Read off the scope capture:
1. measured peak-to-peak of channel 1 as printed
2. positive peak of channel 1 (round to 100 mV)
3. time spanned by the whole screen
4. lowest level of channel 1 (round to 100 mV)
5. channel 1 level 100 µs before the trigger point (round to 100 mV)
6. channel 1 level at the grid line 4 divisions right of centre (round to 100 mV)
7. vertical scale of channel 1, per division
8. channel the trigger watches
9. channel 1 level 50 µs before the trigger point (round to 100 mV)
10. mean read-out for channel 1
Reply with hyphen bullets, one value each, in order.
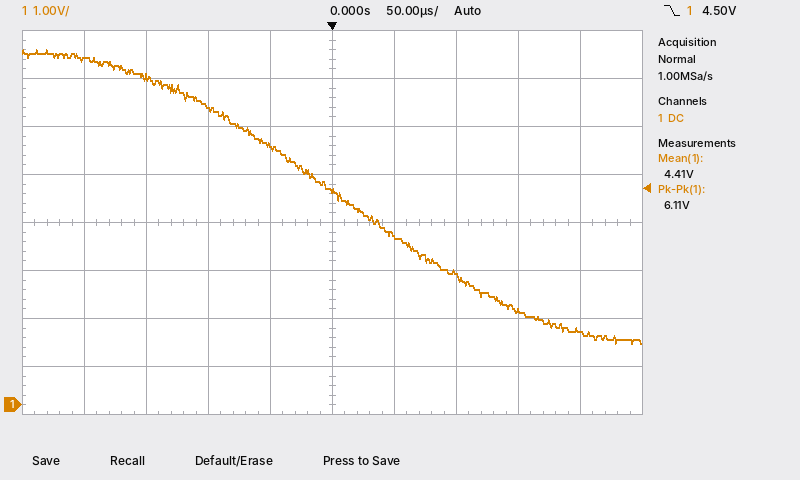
- 6.11 V
- 7.4 V
- 500 µs
- 1.3 V
- 6.2 V
- 1.5 V
- 1 V
- channel 1
- 5.4 V
- 4.41 V
